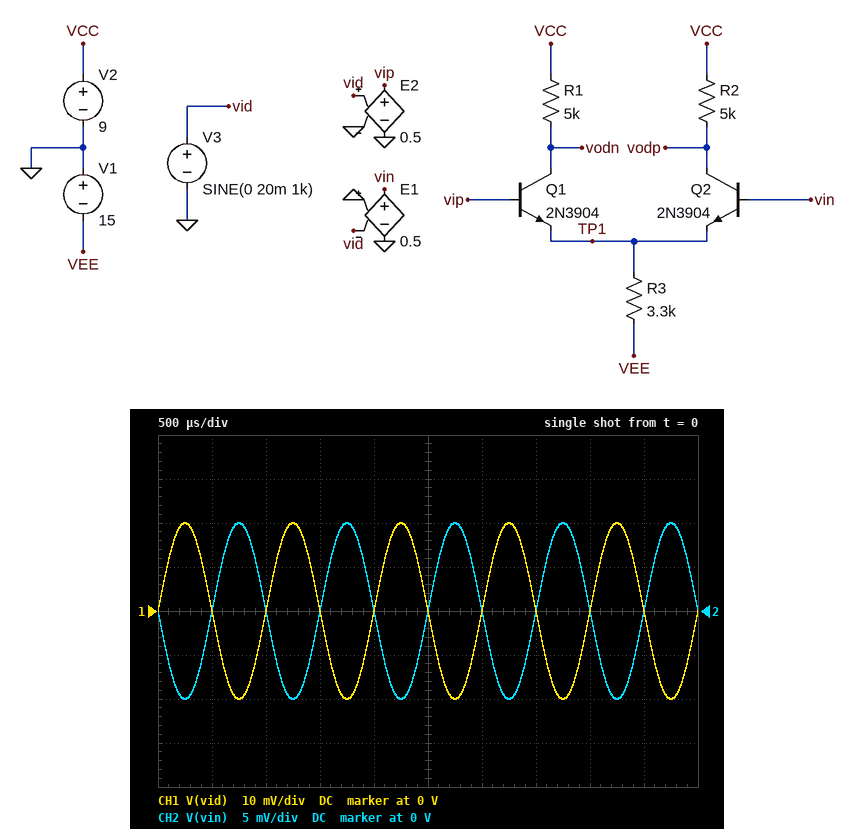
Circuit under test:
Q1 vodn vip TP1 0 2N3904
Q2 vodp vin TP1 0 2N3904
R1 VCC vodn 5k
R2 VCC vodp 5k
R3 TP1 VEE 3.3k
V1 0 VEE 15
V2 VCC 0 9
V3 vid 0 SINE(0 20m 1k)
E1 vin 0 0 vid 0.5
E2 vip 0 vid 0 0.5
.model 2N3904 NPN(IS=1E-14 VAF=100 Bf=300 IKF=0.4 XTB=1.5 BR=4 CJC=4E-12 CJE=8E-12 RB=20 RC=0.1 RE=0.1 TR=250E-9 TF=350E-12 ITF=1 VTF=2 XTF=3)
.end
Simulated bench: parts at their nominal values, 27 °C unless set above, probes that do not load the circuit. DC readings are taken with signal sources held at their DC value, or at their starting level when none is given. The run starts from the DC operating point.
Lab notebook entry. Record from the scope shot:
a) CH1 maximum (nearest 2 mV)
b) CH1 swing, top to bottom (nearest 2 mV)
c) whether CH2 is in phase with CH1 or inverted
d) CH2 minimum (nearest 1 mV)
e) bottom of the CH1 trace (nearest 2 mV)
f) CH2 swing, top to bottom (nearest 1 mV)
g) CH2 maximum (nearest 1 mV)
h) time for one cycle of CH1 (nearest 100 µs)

20 mV
40 mV
inverted
-10 mV
-20 mV
20 mV
10 mV
1.0 ms
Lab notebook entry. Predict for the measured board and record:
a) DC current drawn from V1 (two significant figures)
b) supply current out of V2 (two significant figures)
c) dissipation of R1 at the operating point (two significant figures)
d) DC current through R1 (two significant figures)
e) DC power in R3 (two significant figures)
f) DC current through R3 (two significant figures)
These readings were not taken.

4.3 mA
3.9 mA
19 mW
1.9 mA
62 mW
4.3 mA
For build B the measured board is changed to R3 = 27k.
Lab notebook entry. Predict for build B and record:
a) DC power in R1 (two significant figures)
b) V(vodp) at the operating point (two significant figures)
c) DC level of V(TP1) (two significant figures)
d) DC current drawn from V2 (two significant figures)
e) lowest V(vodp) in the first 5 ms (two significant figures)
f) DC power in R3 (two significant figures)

350 µW
7.7 V
-620 mV
530 µA
7.2 V
7.7 mW
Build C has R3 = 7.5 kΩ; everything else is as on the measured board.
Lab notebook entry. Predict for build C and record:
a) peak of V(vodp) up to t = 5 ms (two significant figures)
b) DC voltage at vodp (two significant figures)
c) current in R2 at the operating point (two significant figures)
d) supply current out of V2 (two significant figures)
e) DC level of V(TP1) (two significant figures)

5.9 V
4.2 V
950 µA
1.9 mA
-650 mV
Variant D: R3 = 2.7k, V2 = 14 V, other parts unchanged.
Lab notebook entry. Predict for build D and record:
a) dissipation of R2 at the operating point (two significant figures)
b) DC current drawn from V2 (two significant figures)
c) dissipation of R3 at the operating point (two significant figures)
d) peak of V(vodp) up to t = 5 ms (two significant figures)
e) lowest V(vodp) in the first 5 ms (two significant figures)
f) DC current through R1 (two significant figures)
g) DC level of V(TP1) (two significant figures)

35 mW
5.3 mA
76 mW
3.2 V
-640 mV
2.6 mA
-680 mV
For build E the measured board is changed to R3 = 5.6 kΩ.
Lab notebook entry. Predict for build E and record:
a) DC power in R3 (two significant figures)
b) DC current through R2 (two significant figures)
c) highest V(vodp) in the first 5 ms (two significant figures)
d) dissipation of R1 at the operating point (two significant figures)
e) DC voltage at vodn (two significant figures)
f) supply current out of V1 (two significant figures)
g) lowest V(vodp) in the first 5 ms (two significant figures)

37 mW
1.3 mA
4.8 V
8.1 mW
2.6 V
2.6 mA
410 mV
